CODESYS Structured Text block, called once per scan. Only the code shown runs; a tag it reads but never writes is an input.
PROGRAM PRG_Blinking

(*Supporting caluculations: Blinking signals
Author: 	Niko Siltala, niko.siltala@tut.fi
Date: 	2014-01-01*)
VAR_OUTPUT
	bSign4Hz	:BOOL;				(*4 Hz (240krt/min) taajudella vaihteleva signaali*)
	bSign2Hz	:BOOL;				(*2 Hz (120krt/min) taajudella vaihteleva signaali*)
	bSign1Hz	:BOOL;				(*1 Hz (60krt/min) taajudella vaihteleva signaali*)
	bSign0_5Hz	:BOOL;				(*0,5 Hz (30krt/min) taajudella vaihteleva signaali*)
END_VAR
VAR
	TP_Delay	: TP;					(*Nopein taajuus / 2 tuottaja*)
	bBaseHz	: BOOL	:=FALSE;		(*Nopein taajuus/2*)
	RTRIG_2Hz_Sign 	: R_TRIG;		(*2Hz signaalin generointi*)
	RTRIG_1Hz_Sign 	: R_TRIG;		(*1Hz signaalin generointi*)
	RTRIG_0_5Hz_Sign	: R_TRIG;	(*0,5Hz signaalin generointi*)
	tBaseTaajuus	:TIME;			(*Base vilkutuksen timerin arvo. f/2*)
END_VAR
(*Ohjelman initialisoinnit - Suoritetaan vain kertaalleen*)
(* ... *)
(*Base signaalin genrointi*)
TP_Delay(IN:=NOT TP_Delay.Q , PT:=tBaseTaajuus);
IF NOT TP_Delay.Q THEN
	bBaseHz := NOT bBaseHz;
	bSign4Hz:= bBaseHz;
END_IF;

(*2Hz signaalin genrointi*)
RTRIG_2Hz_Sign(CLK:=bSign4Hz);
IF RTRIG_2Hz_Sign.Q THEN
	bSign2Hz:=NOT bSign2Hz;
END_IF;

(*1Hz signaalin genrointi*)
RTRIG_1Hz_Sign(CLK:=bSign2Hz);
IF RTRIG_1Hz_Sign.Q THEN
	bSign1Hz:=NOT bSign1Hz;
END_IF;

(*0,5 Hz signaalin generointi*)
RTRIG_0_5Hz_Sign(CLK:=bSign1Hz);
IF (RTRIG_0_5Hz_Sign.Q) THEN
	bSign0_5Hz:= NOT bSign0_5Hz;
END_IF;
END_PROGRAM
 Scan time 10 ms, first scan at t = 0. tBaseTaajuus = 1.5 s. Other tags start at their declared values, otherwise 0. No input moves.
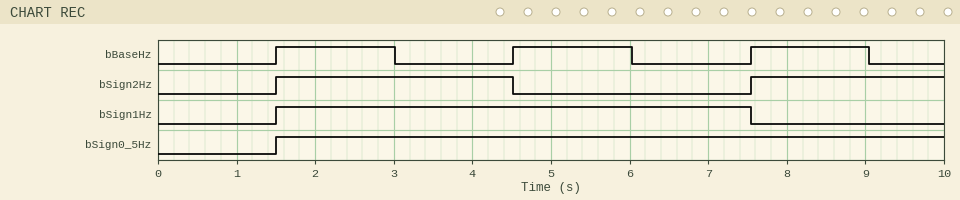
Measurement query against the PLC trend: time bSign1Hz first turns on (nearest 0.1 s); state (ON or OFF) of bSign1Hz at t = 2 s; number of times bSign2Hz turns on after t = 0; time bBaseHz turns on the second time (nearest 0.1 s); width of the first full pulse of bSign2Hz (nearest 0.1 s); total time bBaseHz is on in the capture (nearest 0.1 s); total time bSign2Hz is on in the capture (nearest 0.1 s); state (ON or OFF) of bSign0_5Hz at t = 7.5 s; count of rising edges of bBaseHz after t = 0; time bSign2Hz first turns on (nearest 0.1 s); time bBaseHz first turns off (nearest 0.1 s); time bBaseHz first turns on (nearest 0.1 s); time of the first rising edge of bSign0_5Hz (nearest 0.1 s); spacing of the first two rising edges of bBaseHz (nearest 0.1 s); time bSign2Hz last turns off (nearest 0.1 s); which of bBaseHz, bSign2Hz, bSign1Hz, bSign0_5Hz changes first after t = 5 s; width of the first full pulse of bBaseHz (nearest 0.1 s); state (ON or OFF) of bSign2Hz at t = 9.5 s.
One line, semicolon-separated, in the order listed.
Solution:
1.5 s; ON; 2; 4.5 s; 3.0 s; 4.5 s; 5.5 s; ON; 3; 1.5 s; 3.0 s; 1.5 s; 1.5 s; 3.0 s; 4.5 s; bBaseHz; 1.5 s; ON
